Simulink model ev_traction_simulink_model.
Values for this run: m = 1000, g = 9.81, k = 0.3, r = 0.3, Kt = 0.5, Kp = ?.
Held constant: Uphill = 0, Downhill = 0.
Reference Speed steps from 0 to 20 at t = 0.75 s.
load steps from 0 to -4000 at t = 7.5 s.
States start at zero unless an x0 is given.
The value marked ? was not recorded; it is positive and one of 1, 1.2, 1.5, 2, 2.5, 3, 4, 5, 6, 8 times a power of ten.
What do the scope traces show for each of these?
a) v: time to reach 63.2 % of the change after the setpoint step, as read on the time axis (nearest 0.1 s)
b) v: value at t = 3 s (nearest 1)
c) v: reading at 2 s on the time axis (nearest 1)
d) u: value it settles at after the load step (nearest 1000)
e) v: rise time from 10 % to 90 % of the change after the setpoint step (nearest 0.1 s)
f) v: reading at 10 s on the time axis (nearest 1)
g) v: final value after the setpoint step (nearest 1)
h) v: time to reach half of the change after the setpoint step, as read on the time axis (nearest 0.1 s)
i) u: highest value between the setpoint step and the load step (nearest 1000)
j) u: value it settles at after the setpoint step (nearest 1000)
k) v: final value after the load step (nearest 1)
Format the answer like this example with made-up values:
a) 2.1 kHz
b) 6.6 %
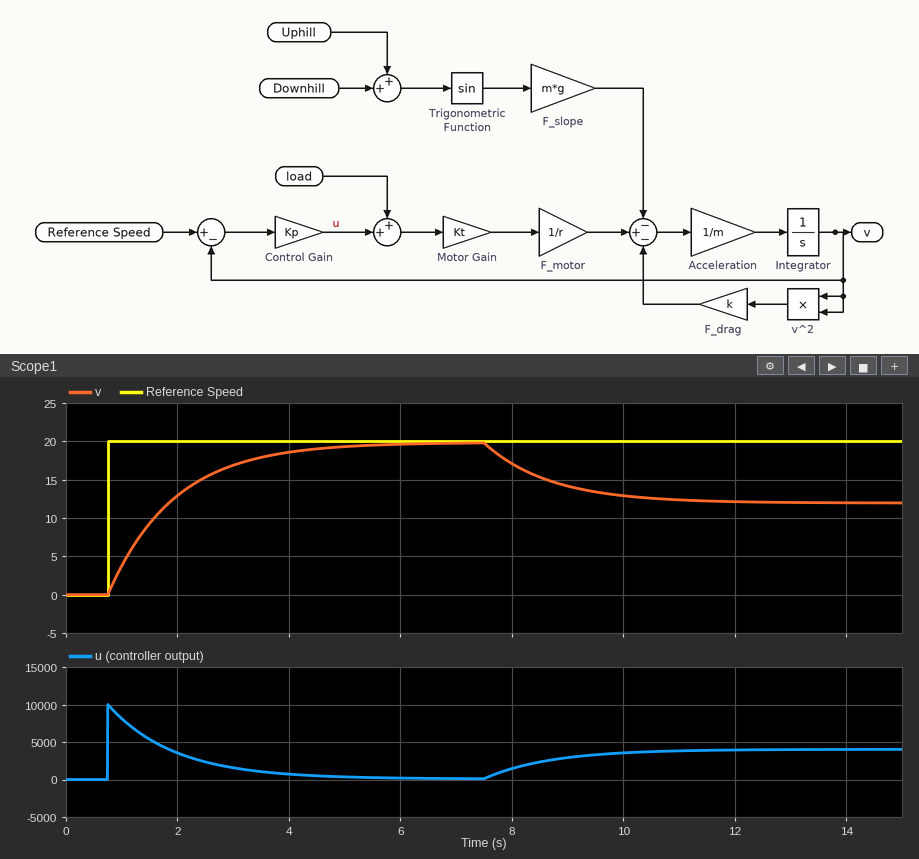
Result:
a) 1.9 s
b) 17
c) 13
d) 4000
e) 2.6 s
f) 13
g) 20
h) 1.6 s
i) 10000
j) 0
k) 12
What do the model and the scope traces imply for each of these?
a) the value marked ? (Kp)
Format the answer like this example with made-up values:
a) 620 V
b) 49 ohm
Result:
a) 500
